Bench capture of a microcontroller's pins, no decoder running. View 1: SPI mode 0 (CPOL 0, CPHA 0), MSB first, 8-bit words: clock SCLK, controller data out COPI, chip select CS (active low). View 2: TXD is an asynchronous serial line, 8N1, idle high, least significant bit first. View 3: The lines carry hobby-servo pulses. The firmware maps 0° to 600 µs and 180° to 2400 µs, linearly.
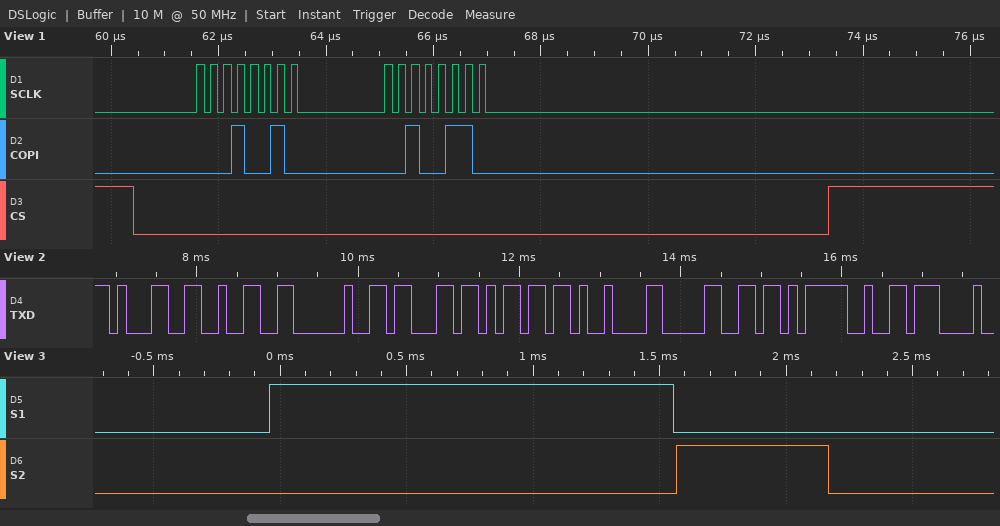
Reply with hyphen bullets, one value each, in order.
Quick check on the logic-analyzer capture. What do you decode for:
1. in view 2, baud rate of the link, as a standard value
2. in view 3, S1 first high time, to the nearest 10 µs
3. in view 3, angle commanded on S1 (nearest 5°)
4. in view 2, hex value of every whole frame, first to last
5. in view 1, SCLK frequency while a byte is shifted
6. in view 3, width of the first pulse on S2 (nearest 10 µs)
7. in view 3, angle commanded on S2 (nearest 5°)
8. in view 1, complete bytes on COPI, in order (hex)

- 9600 baud
- 1600 µs
- 100°
- 31 32 20 63 6D 09 30 EB B2
- 4 MHz
- 600 µs
- 0°
- 12 26
